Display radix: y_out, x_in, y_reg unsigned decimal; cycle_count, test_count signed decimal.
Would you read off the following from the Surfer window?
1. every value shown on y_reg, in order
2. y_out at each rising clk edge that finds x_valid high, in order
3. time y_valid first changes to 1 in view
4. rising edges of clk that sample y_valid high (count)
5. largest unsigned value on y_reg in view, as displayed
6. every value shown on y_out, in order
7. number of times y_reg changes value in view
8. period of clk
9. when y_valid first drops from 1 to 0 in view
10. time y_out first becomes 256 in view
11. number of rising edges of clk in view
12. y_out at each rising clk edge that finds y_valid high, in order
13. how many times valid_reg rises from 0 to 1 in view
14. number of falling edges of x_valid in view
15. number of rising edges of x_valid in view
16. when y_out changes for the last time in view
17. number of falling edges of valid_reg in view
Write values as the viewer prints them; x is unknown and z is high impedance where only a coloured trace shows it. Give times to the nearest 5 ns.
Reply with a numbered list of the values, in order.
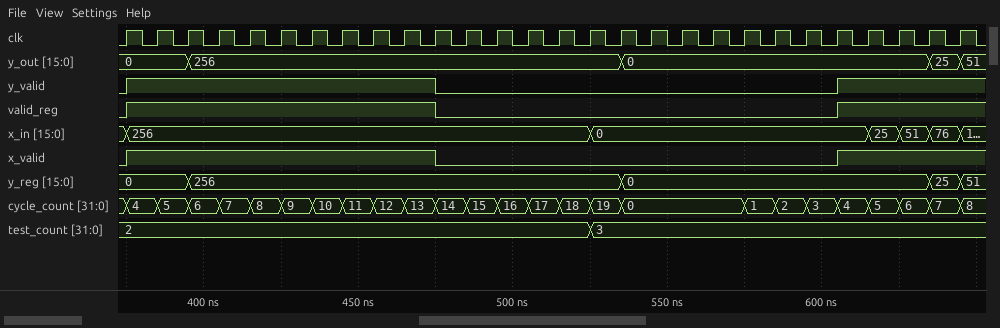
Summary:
1. 0, 256, 0, 25, 51
2. 0, 0, 256, 256, 256, 256, 256, 256, 256, 256, 0, 0, 0, 25
3. 375 ns
4. 14
5. 256
6. 0, 256, 0, 25, 51
7. 4
8. 10 ns
9. 475 ns
10. 395 ns
11. 28
12. 0, 0, 256, 256, 256, 256, 256, 256, 256, 256, 0, 0, 0, 25
13. 2
14. 1
15. 2
16. 645 ns
17. 1
